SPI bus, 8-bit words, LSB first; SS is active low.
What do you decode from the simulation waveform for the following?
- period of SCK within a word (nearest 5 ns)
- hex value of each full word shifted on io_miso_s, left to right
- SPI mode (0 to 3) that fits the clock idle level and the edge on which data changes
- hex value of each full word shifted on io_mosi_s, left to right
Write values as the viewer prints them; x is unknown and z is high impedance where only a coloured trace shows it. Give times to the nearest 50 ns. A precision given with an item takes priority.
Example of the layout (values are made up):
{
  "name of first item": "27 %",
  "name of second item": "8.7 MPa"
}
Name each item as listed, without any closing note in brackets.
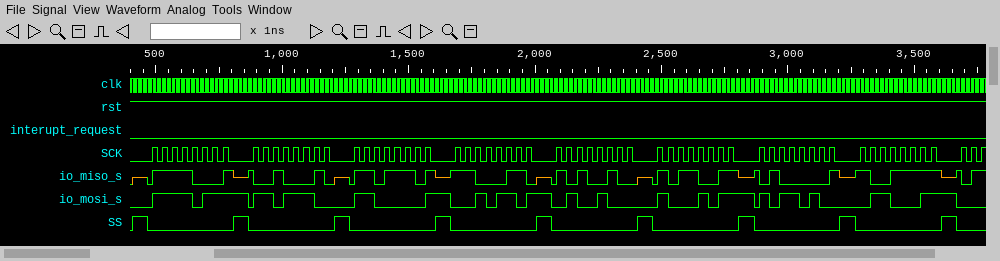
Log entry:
{
  "period of SCK within a word": "40 ns",
  "hex value of each full word shifted on io_miso_s, left to right": "8F, 44, BB, 63, 25, CD, 82, F9",
  "SPI mode (0 to 3) that fits the clock idle level and the edge on which data changes": "1",
  "hex value of each full word shifted on io_mosi_s, left to right": "EF, 3B, 83, B4, 12, D1, 2D, C6"
}
